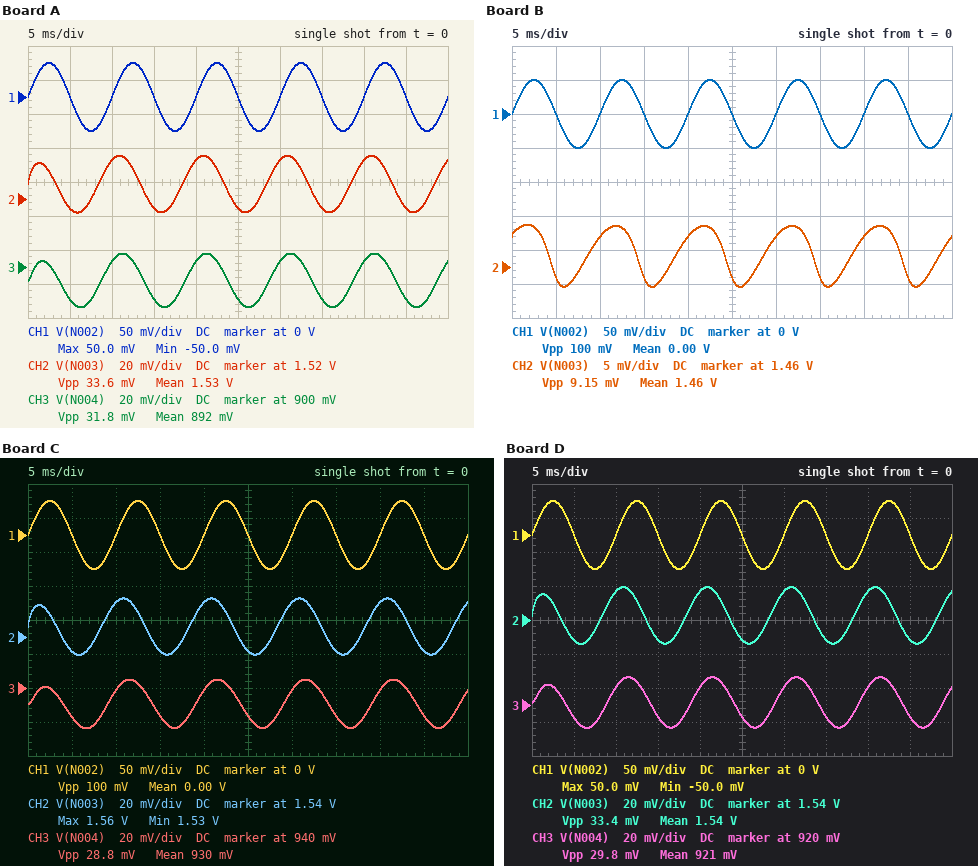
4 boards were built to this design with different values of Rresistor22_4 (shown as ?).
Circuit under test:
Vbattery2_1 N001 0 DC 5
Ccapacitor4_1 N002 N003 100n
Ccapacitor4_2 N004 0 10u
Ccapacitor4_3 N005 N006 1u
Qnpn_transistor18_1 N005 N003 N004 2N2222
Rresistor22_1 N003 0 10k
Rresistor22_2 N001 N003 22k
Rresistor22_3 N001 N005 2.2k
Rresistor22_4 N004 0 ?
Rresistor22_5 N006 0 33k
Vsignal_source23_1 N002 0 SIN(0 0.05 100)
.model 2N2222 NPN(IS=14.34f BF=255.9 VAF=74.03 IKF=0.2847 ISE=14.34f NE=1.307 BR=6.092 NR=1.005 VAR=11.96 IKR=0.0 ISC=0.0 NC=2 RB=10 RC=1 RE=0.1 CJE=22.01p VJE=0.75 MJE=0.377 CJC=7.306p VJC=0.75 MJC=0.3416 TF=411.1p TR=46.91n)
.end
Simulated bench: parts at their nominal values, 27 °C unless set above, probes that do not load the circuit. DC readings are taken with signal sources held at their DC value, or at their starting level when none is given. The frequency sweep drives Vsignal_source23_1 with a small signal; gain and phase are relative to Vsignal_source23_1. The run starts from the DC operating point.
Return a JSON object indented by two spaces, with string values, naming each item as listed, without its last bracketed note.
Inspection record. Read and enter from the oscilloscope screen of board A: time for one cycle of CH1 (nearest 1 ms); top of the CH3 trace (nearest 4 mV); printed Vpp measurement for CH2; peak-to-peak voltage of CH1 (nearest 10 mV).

{
  "time for one cycle of CH1": "10 ms",
  "top of the CH3 trace": "908 mV",
  "printed Vpp measurement for CH2": "33.6 mV",
  "peak-to-peak voltage of CH1": "100 mV"
}
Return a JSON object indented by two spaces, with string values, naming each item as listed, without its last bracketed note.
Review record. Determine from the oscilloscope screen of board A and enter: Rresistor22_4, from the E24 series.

{
  "Rresistor22_4, from the E24 series": "1.3 kΩ"
}
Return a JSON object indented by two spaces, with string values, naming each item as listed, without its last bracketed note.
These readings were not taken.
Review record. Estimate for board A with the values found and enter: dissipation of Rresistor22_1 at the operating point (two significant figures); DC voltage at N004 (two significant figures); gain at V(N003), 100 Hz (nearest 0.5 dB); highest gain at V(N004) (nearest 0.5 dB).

{
  "dissipation of Rresistor22_1 at the operating point": "230 µW",
  "DC voltage at N004": "890 mV",
  "gain at V(N003), 100 Hz": "-9.5 dB",
  "highest gain at V(N004)": "-7.0 dB"
}
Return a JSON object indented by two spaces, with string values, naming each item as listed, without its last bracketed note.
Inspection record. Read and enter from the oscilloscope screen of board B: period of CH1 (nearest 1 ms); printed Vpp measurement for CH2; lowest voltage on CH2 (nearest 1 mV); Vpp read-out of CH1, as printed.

{
  "period of CH1": "10 ms",
  "printed Vpp measurement for CH2": "9.15 mV",
  "lowest voltage on CH2": "1.457 V",
  "Vpp read-out of CH1, as printed": "100 mV"
}
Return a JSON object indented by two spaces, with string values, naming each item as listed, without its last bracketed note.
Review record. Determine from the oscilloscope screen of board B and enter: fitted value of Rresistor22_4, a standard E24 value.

{
  "fitted value of Rresistor22_4, a standard E24 value": "430 Ω"
}
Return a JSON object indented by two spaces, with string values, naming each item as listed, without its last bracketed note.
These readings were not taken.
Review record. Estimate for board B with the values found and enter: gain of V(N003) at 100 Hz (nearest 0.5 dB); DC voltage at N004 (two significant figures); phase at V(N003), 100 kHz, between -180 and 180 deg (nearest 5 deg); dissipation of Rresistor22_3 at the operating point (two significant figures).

{
  "gain of V(N003) at 100 Hz": "-23.5 dB",
  "DC voltage at N004": "800 mV",
  "phase at V(N003), 100 kHz, between -180 and 180 deg": "5 deg",
  "dissipation of Rresistor22_3 at the operating point": "7.5 mW"
}
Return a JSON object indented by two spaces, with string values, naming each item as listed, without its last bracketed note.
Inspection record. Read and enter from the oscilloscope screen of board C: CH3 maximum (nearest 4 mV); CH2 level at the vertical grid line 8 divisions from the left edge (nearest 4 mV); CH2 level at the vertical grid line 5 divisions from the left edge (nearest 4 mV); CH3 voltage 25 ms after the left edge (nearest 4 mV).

{
  "CH3 maximum": "944 mV",
  "CH2 level at the vertical grid line 8 divisions from the left edge": "1.560 V",
  "CH2 level at the vertical grid line 5 divisions from the left edge": "1.532 V",
  "CH3 voltage 25 ms after the left edge": "924 mV"
}
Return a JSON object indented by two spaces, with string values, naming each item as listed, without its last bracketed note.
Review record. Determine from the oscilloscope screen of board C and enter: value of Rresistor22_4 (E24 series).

{
  "value of Rresistor22_4": "3 kΩ"
}
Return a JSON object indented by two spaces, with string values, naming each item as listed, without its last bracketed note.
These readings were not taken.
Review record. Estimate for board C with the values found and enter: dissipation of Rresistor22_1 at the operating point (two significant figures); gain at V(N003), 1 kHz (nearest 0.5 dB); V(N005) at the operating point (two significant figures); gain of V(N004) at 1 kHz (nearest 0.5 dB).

{
  "dissipation of Rresistor22_1 at the operating point": "240 µW",
  "gain at V(N003), 1 kHz": "-0.5 dB",
  "V(N005) at the operating point": "4.3 V",
  "gain of V(N004) at 1 kHz": "-15.5 dB"
}
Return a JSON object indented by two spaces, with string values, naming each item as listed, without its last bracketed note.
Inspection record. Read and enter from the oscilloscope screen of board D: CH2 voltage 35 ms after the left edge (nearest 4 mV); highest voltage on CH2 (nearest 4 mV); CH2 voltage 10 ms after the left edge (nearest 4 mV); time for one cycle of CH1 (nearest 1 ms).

{
  "CH2 voltage 35 ms after the left edge": "1.528 V",
  "highest voltage on CH2": "1.560 V",
  "CH2 voltage 10 ms after the left edge": "1.556 V",
  "time for one cycle of CH1": "10 ms"
}
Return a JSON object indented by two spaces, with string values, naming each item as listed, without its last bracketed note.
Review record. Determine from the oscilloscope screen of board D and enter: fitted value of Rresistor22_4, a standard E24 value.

{
  "fitted value of Rresistor22_4, a standard E24 value": "2.4 kΩ"
}
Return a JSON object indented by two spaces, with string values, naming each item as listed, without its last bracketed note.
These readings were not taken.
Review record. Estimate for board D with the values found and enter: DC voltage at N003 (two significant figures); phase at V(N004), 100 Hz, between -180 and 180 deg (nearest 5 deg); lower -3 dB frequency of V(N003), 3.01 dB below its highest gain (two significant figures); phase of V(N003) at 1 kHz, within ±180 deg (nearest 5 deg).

{
  "DC voltage at N003": "1.5 V",
  "phase at V(N004), 100 Hz, between -180 and 180 deg": "35 deg",
  "lower -3 dB frequency of V(N003), 3.01 dB below its highest gain": "430 Hz",
  "phase of V(N003) at 1 kHz, within ±180 deg": "20 deg"
}
